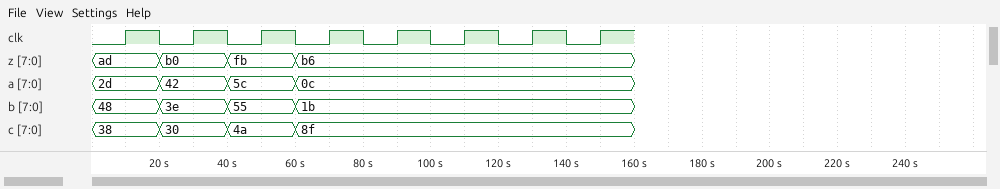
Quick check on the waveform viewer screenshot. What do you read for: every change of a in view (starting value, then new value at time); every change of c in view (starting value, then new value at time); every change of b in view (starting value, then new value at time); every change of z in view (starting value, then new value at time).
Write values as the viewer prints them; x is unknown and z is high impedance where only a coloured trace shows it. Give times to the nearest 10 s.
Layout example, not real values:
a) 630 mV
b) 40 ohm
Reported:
a) 2d, 42 at 20 s, 5c at 40 s, 0c at 60 s
b) 38, 30 at 20 s, 4a at 40 s, 8f at 60 s
c) 48, 3e at 20 s, 55 at 40 s, 1b at 60 s
d) ad, b0 at 20 s, fb at 40 s, b6 at 60 s
